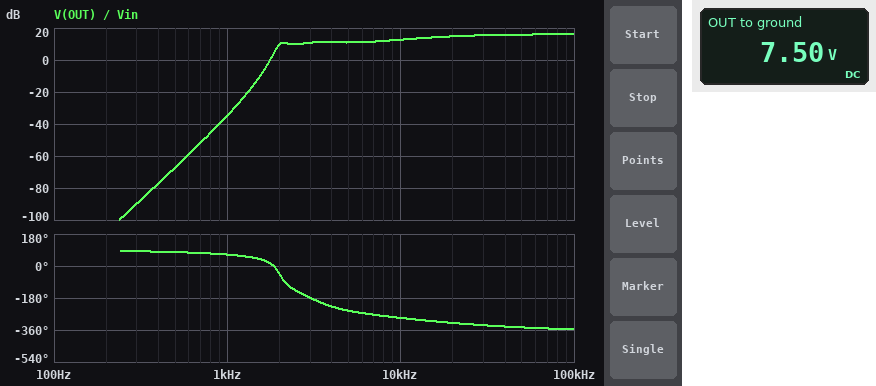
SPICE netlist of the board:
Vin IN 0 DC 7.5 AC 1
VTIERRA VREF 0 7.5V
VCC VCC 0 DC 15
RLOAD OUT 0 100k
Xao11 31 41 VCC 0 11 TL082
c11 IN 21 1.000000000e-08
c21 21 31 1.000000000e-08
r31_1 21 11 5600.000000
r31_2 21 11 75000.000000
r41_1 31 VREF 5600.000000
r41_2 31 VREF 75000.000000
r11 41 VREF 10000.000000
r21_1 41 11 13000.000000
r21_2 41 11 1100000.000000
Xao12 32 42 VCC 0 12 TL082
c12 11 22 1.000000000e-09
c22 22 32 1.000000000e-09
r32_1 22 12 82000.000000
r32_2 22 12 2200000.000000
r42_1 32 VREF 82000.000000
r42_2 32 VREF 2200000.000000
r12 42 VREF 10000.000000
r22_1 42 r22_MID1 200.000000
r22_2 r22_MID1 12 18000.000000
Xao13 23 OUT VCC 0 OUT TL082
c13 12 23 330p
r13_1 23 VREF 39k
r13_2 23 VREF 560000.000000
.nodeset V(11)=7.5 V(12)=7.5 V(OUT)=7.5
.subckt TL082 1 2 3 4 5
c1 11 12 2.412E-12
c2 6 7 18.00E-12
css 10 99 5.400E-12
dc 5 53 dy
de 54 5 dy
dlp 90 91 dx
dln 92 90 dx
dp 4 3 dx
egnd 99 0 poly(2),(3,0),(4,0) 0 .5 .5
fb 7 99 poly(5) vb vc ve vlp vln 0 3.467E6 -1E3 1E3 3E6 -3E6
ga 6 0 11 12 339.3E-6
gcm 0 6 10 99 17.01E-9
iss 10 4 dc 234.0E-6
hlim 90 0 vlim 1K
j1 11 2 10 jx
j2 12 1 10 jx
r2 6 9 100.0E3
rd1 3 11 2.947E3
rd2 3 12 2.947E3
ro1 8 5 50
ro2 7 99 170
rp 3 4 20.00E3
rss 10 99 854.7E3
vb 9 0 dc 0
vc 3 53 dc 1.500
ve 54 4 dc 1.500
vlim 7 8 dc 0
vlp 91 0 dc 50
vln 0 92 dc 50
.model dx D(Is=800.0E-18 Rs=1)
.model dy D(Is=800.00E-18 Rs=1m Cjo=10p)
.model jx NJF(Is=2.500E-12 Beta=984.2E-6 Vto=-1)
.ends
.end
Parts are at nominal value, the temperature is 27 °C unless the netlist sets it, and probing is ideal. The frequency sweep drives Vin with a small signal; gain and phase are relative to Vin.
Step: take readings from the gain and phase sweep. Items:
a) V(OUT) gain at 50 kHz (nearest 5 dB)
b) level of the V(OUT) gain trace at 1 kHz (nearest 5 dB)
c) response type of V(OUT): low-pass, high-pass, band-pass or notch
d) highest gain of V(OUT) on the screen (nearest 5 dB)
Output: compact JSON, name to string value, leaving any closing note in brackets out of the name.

{"V(OUT) gain at 50 kHz": "15 dB", "level of the V(OUT) gain trace at 1 kHz": "-35 dB", "response type of V(OUT): low-pass, high-pass, band-pass or notch": "high-pass", "highest gain of V(OUT) on the screen": "15 dB"}
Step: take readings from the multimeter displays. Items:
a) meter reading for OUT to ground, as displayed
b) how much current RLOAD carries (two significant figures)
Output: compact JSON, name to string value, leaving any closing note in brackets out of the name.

{"meter reading for OUT to ground, as displayed": "7.50 V", "how much current RLOAD carries": "75 µA"}
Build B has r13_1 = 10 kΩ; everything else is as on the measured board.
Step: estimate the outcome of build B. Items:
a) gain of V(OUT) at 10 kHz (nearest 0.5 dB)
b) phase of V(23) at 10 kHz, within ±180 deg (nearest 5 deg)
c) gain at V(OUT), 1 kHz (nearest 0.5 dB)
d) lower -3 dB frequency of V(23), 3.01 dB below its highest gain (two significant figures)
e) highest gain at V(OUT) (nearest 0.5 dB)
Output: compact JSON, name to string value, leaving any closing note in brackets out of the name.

{"gain of V(OUT) at 10 kHz": "3.0 dB", "phase of V(23) at 10 kHz, within ±180 deg": "95 deg", "gain at V(OUT), 1 kHz": "-46.0 dB", "lower -3 dB frequency of V(23), 3.01 dB below its highest gain": "47 kHz", "highest gain at V(OUT)": "16.0 dB"}
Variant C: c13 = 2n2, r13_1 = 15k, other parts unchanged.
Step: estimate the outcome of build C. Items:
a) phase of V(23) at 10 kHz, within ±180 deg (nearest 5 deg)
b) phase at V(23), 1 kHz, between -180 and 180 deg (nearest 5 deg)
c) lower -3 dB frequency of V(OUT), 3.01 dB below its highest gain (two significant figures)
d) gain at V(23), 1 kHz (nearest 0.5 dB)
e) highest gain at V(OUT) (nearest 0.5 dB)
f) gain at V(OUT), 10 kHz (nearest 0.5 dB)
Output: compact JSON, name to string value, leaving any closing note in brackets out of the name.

{"phase of V(23) at 10 kHz, within ±180 deg": "40 deg", "phase at V(23), 1 kHz, between -180 and 180 deg": "55 deg", "lower -3 dB frequency of V(OUT), 3.01 dB below its highest gain": "1.9 kHz", "gain at V(23), 1 kHz": "-26.5 dB", "highest gain at V(OUT)": "18.5 dB", "gain at V(OUT), 10 kHz": "16.0 dB"}
